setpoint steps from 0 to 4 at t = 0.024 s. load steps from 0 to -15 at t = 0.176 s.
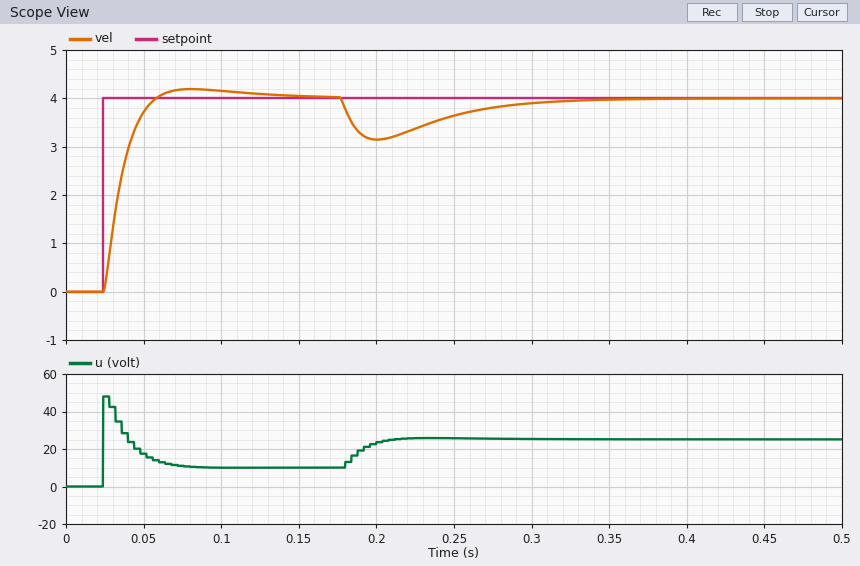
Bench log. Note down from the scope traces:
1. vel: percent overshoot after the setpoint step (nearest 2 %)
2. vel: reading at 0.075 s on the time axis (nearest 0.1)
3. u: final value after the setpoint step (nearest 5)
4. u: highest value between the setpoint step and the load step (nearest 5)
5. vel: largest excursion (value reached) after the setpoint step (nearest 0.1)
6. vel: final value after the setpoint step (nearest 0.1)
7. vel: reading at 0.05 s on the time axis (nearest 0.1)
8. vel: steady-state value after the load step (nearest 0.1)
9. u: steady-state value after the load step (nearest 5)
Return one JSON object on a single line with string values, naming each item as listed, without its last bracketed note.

{"vel: percent overshoot after the setpoint step": "4 %", "vel: reading at 0.075 s on the time axis": "4.2", "u: final value after the setpoint step": "10", "u: highest value between the setpoint step and the load step": "50", "vel: largest excursion (value reached) after the setpoint step": "4.2", "vel: final value after the setpoint step": "4.0", "vel: reading at 0.05 s on the time axis": "3.7", "vel: steady-state value after the load step": "4.0", "u: steady-state value after the load step": "25"}
